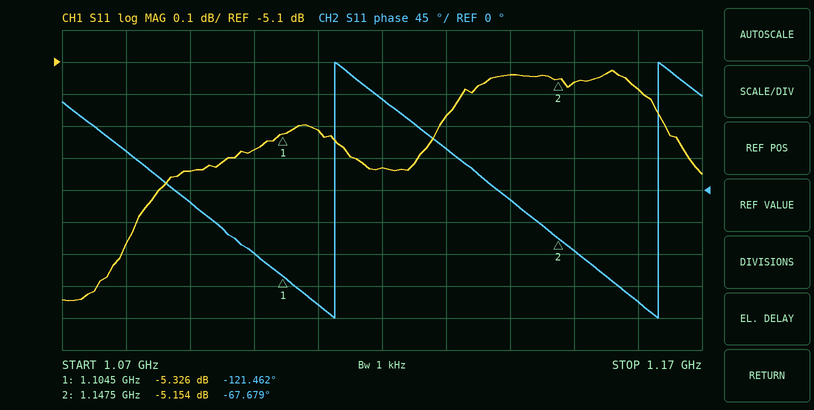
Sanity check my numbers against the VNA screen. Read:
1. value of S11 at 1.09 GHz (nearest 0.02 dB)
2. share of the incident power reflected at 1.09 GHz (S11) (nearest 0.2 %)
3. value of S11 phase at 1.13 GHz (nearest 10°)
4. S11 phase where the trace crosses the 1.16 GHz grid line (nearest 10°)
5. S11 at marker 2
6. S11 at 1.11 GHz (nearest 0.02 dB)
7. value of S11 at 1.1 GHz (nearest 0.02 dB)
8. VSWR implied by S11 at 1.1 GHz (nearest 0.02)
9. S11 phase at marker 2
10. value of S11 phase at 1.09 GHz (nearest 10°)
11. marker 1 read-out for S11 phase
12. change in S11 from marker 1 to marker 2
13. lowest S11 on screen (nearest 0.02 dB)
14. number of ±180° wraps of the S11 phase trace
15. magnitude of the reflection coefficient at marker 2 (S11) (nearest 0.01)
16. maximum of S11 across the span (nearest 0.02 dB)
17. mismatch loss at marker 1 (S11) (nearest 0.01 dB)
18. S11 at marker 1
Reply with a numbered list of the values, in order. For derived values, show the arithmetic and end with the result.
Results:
1. -5.44 dB
2. 10^(-5.44/10) ≈ 28.6 %
3. 60°
4. -160°
5. -5.154 dB
6. -5.32 dB
7. -5.38 dB
8. |Γ| = 10^(-5.38/20) = 0.5383; VSWR = (1 + 0.5383)/(1 − 0.5383) ≈ 3.33, so 3.34 to the nearest 0.02
9. -67.679°
10. -20°
11. -121.462°
12. -5.154 − (-5.326) = 0.172 dB
13. -5.84 dB
14. 2
15. 10^(-5.154/20) ≈ 0.55
16. -5.12 dB
17. −10 log10(1 − 10^(-5.326/10)) ≈ 1.51 dB
18. -5.326 dB
